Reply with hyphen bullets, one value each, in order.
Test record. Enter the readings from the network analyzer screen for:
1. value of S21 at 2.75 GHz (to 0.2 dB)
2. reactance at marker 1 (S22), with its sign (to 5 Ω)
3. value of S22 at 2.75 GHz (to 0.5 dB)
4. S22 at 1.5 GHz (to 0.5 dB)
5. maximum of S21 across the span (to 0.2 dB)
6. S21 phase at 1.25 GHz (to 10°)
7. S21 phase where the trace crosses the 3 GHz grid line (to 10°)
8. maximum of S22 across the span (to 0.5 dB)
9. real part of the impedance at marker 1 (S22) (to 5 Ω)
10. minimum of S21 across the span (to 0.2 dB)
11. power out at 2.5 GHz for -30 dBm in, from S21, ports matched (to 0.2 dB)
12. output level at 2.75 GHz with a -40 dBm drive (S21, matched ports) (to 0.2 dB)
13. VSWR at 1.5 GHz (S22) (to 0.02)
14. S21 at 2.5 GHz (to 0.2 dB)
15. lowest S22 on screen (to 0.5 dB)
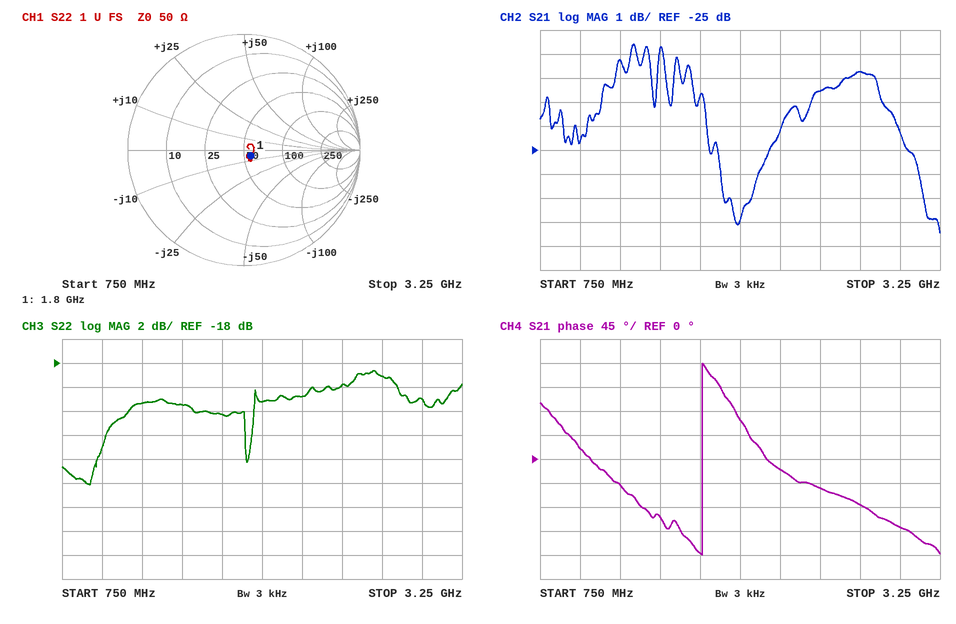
- -21.8 dB
- -5 Ω
- -19.0 dB
- -21.5 dB
- -20.6 dB
- -50°
- -130°
- -18.5 dB
- 55 Ω
- -28.4 dB
- -52.6 dBm
- -61.8 dBm
- 1.18
- -22.6 dB
- -28.0 dB
